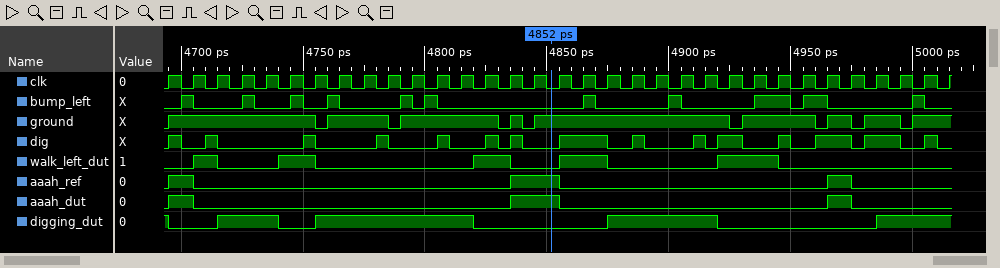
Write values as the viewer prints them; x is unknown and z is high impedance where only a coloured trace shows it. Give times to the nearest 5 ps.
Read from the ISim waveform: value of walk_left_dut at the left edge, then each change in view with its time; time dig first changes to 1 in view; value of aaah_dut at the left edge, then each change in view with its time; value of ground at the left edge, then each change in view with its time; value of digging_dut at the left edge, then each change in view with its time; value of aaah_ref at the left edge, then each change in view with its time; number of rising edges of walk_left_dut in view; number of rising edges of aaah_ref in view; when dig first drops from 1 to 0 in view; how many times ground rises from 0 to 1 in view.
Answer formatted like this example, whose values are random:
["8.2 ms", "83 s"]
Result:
["0, 1 at 4705 ps, 0 at 4715 ps, 1 at 4740 ps, 0 at 4755 ps, 1 at 4820 ps, 0 at 4835 ps, 1 at 4855 ps, 0 at 4875 ps, 1 at 4920 ps, 0 at 4945 ps", "4695 ps", "0, 1 at 4695 ps, 0 at 4705 ps, 1 at 4835 ps, 0 at 4855 ps, 1 at 4965 ps, 0 at 4975 ps", "0, 1 at 4695 ps, 0 at 4755 ps, 1 at 4760 ps, 0 at 4785 ps, 1 at 4790 ps, 0 at 4830 ps, 1 at 4835 ps, 0 at 4840 ps, 1 at 4845 ps, 0 at 4925 ps, 1 at 4930 ps, 0 at 4960 ps, 1 at 4965 ps, 0 at 4975 ps, 1 at 4980 ps, 0 at 4995 ps, 1 at 5000 ps", "1, 0 at 4695 ps, 1 at 4715 ps, 0 at 4740 ps, 1 at 4755 ps, 0 at 4820 ps, 1 at 4875 ps, 0 at 4920 ps, 1 at 4985 ps", "0, 1 at 4695 ps, 0 at 4705 ps, 1 at 4835 ps, 0 at 4855 ps, 1 at 4965 ps, 0 at 4975 ps", "5", "3", "4700 ps", "9"]
